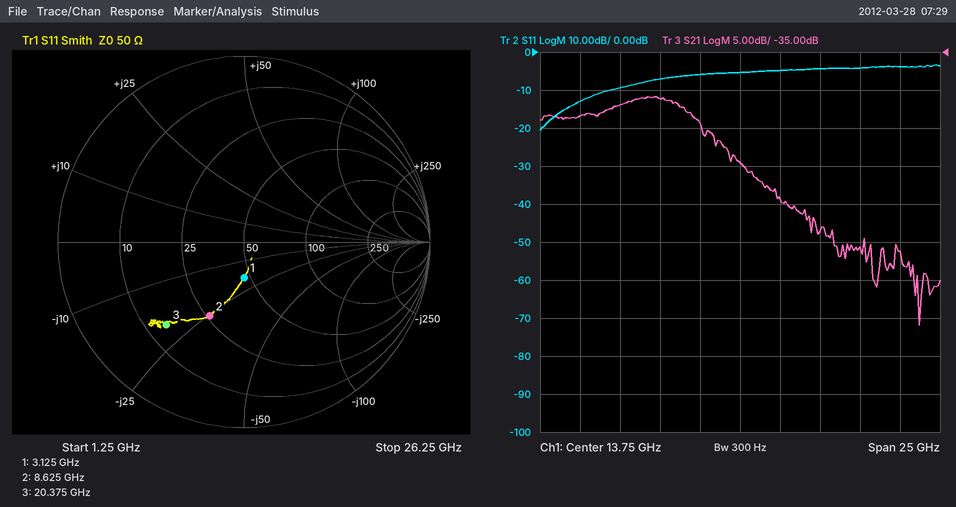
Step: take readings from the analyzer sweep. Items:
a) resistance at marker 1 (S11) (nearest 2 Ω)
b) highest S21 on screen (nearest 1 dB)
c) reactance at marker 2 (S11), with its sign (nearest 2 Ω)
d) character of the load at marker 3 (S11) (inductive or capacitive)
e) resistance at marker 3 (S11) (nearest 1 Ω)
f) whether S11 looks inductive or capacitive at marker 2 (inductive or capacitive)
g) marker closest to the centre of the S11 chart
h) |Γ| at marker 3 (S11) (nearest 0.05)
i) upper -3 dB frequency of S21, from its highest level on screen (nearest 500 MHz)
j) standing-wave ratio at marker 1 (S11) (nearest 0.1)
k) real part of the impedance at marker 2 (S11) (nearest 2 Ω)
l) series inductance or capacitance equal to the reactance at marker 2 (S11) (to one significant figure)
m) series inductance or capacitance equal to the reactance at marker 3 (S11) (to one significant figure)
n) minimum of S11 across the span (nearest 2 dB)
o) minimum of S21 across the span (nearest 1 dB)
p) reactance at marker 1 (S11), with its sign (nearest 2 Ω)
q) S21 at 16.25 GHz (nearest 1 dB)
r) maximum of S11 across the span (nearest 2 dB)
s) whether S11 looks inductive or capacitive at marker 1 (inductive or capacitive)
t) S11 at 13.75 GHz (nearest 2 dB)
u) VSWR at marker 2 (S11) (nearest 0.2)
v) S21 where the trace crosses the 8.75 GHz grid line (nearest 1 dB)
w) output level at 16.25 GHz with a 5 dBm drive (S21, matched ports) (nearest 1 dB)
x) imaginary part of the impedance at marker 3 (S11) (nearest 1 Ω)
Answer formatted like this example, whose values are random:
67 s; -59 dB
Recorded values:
46 Ω; -41 dB; -26 Ω; capacitive; 14 Ω; capacitive; marker 1; 0.60; 11.0 GHz; 1.5; 26 Ω; 700 fF; 400 fF; -20 dB; -71 dB; -18 Ω; -54 dB; -4 dB; capacitive; -6 dB; 2.6; -41 dB; -49 dBm; -20 Ω
